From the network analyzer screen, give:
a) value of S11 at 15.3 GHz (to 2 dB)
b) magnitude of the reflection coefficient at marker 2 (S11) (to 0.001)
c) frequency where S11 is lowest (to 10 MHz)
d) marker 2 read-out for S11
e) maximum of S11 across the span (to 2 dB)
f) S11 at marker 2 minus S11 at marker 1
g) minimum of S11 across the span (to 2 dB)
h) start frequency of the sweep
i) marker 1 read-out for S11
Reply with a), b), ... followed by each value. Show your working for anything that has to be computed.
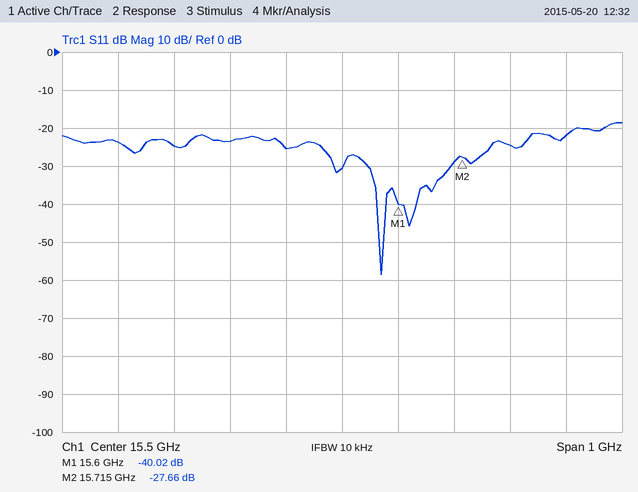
a) -24 dB
b) 10^(-27.66/20) ≈ 0.041
c) 15.57 GHz
d) -27.66 dB
e) -18 dB
f) -27.66 − (-40.02) = 12.36 dB
g) -58 dB
h) 15 GHz
i) -40.02 dB
